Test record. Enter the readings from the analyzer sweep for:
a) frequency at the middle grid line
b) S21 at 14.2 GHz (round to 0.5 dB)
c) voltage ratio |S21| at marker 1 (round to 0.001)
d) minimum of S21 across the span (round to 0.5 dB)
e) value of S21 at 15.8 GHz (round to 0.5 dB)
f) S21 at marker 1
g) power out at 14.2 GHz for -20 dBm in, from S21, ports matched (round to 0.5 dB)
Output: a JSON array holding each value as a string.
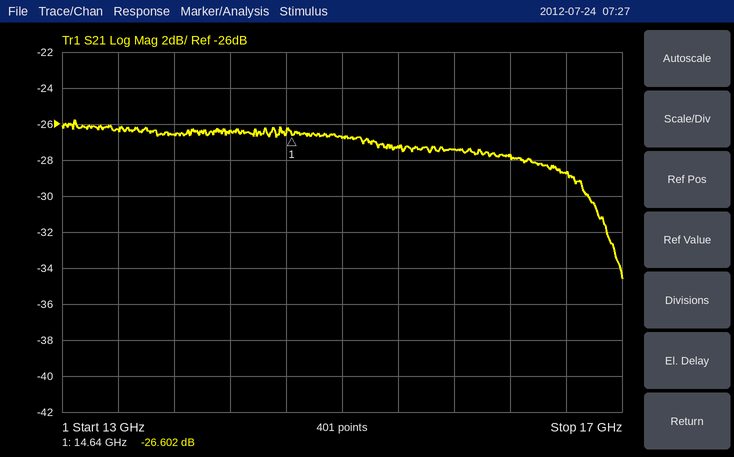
["15 GHz", "-26.5 dB", "0.047", "-34.5 dB", "-27.5 dB", "-26.602 dB", "-46.5 dBm"]
